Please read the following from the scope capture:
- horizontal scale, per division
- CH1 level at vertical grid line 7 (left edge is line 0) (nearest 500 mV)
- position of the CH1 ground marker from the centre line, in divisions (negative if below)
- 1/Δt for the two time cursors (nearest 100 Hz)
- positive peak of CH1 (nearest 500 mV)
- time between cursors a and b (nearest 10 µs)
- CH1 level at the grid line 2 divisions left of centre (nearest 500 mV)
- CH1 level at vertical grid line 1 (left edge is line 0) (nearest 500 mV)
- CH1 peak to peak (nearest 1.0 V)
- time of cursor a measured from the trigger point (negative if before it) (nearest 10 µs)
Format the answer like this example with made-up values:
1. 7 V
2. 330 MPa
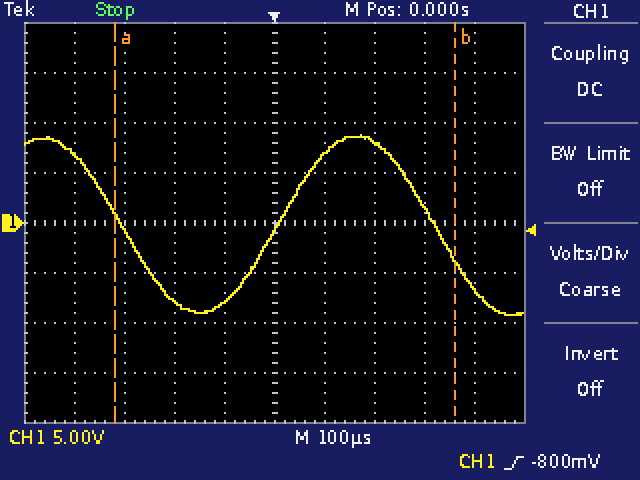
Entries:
1. 100 µs
2. 8.0 V
3. 0.0 div
4. 1.5 kHz
5. 9.0 V
6. 680 µs
7. -8.0 V
8. 7.0 V
9. 18.0 V
10. -320 µs
